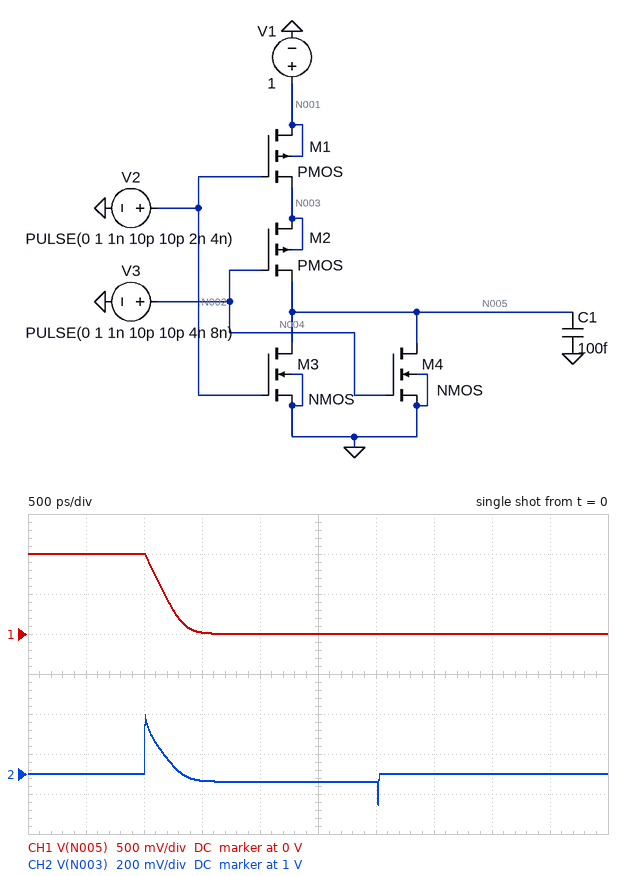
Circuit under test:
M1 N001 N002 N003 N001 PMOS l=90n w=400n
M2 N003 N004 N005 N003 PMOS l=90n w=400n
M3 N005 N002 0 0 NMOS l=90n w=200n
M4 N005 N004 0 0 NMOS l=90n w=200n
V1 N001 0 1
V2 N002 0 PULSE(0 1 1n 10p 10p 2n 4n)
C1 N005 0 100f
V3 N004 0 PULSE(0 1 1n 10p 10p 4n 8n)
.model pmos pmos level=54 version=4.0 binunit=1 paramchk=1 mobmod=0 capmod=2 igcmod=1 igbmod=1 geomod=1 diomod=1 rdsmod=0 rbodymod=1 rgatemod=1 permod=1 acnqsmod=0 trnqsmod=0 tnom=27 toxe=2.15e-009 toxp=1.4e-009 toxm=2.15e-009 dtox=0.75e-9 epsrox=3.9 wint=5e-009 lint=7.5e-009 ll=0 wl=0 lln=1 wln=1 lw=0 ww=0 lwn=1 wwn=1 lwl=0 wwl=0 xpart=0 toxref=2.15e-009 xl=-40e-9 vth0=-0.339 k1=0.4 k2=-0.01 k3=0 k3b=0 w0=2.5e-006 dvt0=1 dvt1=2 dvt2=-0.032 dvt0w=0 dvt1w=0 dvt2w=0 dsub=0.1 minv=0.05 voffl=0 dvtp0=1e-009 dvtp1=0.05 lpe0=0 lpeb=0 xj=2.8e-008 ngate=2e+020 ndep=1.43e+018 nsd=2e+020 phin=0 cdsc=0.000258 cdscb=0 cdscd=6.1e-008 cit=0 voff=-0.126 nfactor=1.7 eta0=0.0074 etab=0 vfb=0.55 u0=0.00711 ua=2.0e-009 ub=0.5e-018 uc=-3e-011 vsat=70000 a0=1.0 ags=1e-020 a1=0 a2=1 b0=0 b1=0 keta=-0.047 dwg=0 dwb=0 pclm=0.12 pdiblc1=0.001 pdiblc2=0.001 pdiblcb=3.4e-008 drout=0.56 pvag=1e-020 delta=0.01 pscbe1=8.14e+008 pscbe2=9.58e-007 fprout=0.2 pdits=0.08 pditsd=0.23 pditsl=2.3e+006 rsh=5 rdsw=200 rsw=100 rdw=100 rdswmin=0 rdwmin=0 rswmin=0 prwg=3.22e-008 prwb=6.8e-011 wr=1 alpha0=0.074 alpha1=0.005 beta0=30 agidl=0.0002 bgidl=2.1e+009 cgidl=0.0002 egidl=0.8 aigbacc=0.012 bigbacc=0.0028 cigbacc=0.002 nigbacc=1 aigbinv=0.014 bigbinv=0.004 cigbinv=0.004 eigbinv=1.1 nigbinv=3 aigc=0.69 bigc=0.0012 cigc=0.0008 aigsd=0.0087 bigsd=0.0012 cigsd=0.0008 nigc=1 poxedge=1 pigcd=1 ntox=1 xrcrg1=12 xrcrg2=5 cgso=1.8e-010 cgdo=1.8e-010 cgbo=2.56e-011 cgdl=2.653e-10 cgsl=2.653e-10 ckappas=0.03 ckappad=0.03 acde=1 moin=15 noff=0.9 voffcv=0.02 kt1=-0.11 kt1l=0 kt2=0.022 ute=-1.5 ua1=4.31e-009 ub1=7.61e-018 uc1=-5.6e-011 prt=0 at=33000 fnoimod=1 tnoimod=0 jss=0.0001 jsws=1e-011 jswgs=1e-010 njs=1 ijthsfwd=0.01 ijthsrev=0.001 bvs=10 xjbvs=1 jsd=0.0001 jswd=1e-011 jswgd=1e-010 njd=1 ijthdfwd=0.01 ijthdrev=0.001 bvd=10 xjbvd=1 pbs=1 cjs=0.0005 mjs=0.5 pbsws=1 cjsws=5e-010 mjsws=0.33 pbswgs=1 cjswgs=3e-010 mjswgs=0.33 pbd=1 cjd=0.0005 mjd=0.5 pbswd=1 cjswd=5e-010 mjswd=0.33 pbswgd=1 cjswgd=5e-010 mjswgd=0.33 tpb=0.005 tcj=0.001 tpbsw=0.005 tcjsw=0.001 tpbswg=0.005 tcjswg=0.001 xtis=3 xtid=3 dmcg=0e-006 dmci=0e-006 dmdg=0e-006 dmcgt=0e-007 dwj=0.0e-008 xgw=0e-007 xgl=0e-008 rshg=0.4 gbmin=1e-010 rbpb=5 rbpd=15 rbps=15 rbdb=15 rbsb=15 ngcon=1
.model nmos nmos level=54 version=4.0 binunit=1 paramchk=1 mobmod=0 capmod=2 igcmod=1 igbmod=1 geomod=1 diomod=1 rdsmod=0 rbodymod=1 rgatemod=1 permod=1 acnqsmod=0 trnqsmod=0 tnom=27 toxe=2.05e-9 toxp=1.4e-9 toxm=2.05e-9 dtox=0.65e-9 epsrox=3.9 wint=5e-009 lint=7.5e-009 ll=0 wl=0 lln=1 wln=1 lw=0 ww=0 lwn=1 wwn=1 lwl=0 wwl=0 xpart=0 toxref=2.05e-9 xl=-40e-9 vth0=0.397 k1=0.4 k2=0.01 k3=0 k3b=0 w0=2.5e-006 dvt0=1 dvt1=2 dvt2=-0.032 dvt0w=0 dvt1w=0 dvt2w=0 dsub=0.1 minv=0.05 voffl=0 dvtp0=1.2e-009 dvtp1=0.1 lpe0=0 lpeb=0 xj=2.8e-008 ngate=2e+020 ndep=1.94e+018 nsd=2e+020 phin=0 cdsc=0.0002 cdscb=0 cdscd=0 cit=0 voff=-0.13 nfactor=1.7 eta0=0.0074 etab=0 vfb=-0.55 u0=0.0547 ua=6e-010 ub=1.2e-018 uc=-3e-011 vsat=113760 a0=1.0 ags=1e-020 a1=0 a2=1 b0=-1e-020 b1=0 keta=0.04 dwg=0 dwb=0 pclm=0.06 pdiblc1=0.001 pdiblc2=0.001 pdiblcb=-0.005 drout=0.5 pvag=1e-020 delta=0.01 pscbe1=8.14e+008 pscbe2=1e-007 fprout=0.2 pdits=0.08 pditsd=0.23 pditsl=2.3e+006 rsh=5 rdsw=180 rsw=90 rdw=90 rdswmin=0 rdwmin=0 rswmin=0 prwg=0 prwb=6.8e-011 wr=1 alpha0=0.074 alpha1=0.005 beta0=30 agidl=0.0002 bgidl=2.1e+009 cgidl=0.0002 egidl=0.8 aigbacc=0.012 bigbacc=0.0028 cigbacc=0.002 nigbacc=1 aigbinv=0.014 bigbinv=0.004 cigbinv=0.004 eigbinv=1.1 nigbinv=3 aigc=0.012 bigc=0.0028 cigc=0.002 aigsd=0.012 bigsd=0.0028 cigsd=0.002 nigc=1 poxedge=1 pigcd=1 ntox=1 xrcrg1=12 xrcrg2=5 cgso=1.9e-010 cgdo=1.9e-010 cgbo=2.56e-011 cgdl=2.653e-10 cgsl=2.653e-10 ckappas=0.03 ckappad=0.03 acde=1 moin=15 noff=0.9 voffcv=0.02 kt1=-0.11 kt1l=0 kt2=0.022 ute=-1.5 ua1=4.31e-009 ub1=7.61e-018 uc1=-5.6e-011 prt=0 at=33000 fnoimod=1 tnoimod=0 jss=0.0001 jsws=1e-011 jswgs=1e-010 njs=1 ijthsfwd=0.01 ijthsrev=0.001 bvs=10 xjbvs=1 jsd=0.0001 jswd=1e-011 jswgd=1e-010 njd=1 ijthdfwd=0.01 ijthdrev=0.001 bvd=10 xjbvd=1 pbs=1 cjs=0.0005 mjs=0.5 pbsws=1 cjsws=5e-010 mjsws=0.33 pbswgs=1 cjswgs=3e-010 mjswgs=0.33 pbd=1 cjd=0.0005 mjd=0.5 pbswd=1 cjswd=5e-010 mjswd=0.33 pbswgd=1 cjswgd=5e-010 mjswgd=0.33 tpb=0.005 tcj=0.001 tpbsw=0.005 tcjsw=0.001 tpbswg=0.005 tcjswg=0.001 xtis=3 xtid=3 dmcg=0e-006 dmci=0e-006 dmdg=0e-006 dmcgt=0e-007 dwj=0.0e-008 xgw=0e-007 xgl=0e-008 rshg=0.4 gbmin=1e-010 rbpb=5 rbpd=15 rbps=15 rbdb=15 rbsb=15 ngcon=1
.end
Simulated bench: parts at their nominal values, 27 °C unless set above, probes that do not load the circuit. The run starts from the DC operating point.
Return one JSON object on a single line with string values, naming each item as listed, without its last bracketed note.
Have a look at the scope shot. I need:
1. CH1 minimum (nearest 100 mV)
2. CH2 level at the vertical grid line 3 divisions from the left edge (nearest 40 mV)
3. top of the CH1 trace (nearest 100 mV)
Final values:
{"CH1 minimum": "0 V", "CH2 level at the vertical grid line 3 divisions from the left edge": "960 mV", "top of the CH1 trace": "1.0 V"}
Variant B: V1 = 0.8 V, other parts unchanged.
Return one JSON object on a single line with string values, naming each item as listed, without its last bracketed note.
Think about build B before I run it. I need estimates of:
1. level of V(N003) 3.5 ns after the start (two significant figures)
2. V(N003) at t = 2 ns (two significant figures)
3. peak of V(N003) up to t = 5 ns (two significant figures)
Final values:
{"level of V(N003) 3.5 ns after the start": "800 mV", "V(N003) at t = 2 ns": "940 mV", "peak of V(N003) up to t = 5 ns": "1.2 V"}
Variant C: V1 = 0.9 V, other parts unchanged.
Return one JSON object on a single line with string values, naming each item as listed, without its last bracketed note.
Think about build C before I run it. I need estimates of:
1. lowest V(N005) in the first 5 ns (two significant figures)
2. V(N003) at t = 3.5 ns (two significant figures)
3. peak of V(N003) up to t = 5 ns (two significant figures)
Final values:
{"lowest V(N005) in the first 5 ns": "-1.7 mV", "V(N003) at t = 3.5 ns": "900 mV", "peak of V(N003) up to t = 5 ns": "1.2 V"}
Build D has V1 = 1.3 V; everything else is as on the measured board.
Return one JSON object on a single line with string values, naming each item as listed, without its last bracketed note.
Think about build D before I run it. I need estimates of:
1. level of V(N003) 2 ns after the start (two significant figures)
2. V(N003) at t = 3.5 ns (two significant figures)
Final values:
{"level of V(N003) 2 ns after the start": "1.2 V", "V(N003) at t = 3.5 ns": "1.3 V"}
